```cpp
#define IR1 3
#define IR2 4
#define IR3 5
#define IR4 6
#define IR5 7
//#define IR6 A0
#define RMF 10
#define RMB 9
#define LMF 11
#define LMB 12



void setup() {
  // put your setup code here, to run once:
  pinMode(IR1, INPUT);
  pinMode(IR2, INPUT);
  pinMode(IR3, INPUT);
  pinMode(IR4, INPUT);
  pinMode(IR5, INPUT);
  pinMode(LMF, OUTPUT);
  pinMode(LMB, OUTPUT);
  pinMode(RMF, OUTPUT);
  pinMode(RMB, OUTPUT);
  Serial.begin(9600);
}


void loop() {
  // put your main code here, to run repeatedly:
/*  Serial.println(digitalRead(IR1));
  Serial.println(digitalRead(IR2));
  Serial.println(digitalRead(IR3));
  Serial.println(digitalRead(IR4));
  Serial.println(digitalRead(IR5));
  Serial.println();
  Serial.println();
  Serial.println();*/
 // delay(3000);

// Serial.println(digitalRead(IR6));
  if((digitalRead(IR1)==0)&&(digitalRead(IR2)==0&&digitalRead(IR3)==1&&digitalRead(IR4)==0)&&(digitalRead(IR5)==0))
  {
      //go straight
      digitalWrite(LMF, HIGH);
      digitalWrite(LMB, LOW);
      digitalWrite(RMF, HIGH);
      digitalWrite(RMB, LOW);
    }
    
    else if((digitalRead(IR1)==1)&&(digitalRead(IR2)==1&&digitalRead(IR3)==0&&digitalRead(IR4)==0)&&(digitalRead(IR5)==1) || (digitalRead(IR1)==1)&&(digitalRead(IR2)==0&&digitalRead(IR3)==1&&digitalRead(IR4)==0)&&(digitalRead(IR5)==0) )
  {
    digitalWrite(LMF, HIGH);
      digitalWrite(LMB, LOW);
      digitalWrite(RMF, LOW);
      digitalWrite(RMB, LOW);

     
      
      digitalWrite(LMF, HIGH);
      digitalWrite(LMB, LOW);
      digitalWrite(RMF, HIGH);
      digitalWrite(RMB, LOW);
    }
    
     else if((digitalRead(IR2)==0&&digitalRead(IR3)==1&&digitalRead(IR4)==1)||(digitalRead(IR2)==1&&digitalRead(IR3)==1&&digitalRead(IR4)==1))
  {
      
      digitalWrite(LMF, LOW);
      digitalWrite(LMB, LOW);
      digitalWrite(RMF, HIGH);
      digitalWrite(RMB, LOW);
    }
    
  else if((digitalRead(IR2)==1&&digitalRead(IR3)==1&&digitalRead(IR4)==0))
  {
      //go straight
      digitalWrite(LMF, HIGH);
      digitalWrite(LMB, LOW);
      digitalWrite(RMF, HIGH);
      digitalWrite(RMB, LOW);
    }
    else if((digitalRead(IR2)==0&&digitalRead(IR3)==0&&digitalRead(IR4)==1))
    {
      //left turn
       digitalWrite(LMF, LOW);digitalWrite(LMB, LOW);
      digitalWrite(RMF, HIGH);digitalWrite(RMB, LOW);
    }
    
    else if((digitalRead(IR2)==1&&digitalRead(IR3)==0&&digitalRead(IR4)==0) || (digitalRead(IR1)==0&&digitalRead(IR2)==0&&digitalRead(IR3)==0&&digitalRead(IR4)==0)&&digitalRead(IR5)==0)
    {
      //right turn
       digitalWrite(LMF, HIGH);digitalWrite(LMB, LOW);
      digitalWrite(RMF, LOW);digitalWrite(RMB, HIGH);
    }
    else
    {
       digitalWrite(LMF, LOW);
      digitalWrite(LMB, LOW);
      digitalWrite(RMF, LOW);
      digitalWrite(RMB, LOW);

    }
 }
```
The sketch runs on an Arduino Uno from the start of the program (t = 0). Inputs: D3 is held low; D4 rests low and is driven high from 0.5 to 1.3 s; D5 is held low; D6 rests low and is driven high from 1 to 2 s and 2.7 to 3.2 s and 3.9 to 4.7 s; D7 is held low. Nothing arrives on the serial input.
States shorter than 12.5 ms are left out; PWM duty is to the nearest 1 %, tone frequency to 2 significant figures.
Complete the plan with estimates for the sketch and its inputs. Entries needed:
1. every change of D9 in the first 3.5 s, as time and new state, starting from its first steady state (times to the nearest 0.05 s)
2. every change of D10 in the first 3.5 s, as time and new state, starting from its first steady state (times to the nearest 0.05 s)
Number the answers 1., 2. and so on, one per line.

1. 0 s high; 1 s low; 2 s high; 2.7 s low; 3.2 s high
2. 0 s low; 1.3 s high; 2 s low; 2.7 s high; 3.2 s low
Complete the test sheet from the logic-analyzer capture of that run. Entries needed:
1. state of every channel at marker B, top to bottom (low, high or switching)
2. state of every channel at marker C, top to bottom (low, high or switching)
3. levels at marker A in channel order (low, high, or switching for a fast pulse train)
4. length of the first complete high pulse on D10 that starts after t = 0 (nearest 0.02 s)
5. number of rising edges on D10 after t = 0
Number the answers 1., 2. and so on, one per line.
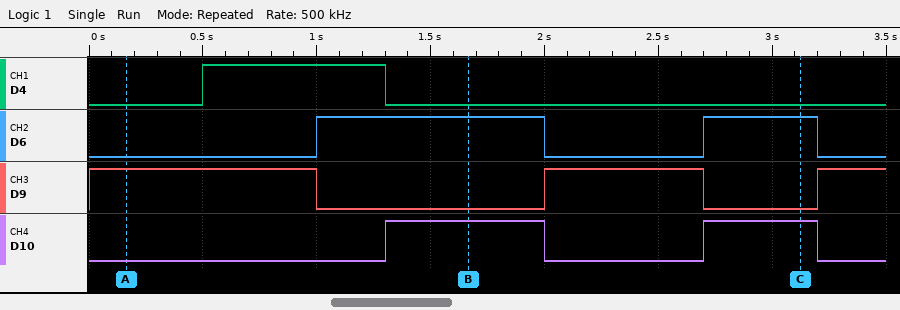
1. D4 low, D6 high, D9 low, D10 high
2. D4 low, D6 high, D9 low, D10 high
3. D4 low, D6 low, D9 high, D10 low
4. 0.70 s
5. 2
